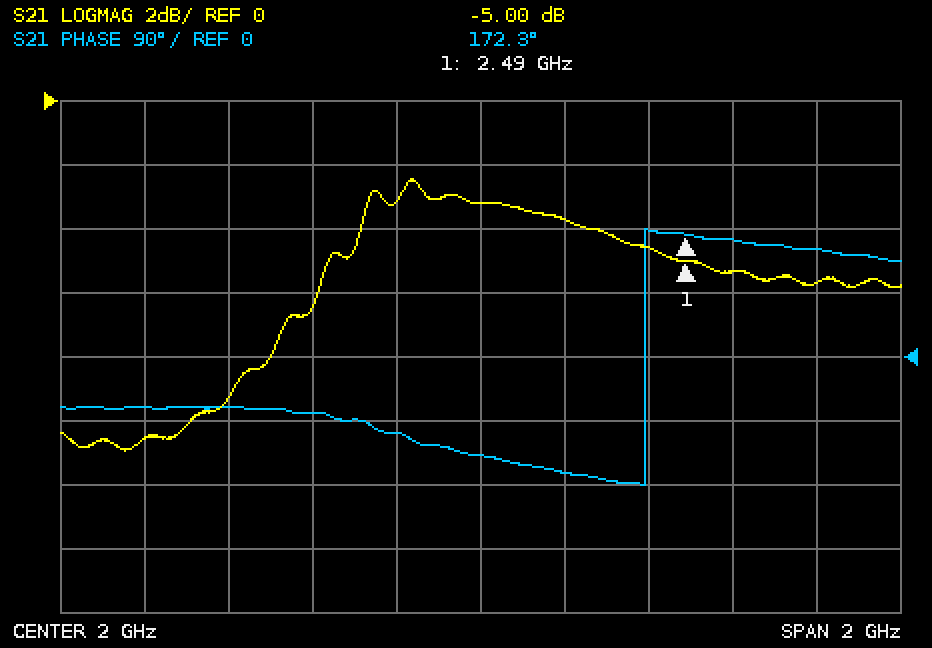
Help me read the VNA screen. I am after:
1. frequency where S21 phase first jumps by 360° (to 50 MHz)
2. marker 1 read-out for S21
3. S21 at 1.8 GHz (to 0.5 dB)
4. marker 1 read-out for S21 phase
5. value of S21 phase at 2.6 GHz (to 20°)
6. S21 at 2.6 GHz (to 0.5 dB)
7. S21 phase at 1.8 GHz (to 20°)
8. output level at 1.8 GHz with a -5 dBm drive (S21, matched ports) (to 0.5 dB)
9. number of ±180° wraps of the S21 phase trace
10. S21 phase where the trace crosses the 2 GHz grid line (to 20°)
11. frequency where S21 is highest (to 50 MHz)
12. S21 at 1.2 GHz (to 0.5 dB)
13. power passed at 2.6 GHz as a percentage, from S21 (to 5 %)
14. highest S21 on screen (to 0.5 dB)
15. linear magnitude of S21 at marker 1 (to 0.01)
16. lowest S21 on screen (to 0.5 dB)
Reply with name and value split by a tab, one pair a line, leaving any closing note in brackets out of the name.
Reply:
frequency where S21 phase first jumps by 360°	2.40 GHz
marker 1 read-out for S21	-5.00 dB
S21 at 1.8 GHz	-3.0 dB
marker 1 read-out for S21 phase	172.3°
value of S21 phase at 2.6 GHz	160°
S21 at 2.6 GHz	-5.5 dB
S21 phase at 1.8 GHz	-100°
output level at 1.8 GHz with a -5 dBm drive (S21, matched ports)	-8.0 dBm
number of ±180° wraps of the S21 phase trace	1
S21 phase where the trace crosses the 2 GHz grid line	-140°
frequency where S21 is highest	1.85 GHz
S21 at 1.2 GHz	-10.5 dB
power passed at 2.6 GHz as a percentage, from S21	30 %
highest S21 on screen	-2.5 dB
linear magnitude of S21 at marker 1	0.56
lowest S21 on screen	-11.0 dB
